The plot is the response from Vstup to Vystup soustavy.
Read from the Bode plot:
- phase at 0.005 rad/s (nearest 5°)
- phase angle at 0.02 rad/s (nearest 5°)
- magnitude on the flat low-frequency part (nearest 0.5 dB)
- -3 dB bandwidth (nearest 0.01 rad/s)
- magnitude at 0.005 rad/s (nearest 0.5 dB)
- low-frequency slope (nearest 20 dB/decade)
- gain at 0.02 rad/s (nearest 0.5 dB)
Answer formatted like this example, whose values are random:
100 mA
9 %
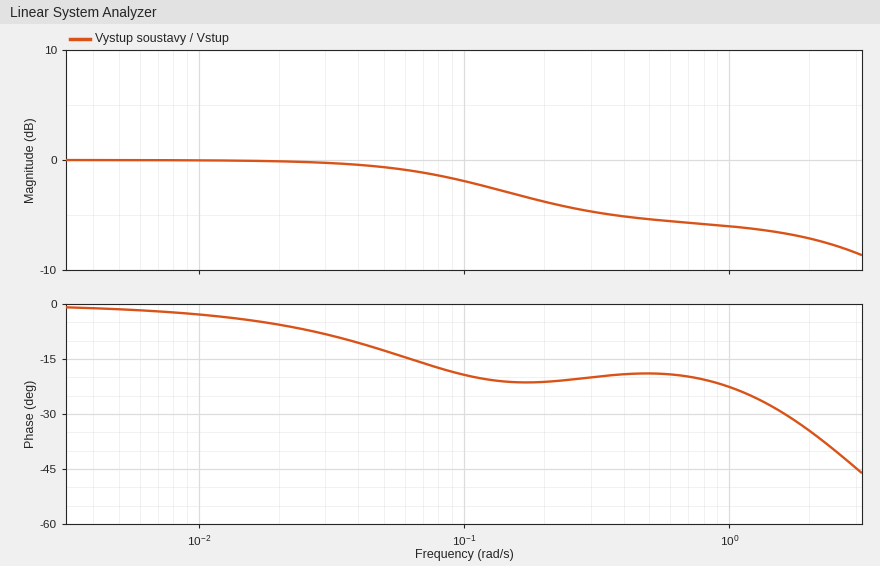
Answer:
0°
-5°
0.0 dB
0.15 rad/s
0.0 dB
0 dB/decade
0.0 dB
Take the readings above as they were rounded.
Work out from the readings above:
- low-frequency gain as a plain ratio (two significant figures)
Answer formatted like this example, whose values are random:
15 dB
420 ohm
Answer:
1.0
